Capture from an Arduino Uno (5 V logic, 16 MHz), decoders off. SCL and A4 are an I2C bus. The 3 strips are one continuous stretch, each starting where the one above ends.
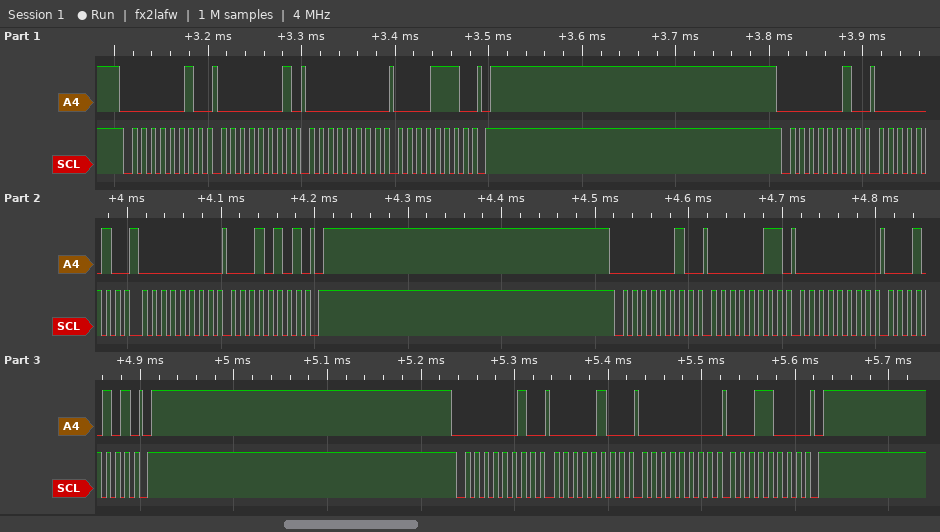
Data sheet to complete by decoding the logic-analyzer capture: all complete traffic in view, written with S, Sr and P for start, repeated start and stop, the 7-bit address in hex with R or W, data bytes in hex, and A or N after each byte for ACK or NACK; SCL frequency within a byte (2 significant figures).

S 01W A 01 A 00 A 0E A P S 01W A 02 A 00 A 15 A P S 01W A 03 A 00 A 15 A P S 01W A 04 A 00 A 18 A P
100 kHz
